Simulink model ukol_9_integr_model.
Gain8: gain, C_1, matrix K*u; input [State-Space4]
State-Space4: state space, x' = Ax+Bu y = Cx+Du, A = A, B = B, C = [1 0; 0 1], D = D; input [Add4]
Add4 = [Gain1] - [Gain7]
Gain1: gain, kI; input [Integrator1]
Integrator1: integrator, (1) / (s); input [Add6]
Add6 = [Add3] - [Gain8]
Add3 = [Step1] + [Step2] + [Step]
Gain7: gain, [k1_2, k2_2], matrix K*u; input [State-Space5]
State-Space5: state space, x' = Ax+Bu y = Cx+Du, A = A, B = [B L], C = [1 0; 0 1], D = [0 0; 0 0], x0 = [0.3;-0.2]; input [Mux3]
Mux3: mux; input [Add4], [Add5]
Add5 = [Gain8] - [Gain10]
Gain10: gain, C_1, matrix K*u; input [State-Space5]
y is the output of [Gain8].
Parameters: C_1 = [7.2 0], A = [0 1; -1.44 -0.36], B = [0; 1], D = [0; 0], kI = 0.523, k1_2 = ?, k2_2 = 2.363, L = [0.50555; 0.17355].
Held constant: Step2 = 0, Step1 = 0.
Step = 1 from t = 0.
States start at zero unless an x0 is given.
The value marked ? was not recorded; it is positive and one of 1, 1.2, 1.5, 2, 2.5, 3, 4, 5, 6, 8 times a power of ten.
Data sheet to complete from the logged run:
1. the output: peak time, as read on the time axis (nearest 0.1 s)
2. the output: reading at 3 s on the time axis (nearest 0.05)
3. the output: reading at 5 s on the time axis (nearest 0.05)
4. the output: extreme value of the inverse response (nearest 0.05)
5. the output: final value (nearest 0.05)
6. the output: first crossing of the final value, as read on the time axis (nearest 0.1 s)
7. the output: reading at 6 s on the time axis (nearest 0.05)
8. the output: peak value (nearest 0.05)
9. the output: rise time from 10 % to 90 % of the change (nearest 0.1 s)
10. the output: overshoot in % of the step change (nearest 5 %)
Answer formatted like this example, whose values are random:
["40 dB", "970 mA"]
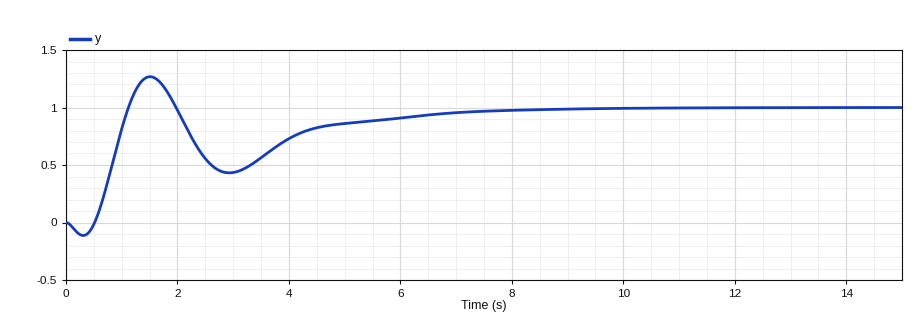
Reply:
["1.5 s", "0.45", "0.85", "-0.10", "1.00", "1.1 s", "0.90", "1.25", "0.5 s", "25 %"]
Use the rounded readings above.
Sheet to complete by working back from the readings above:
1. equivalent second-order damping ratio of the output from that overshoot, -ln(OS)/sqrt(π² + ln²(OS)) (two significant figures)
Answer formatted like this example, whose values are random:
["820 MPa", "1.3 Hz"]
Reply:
["0.40"]
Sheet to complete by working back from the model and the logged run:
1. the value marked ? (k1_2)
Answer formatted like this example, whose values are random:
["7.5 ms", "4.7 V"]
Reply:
["6"]
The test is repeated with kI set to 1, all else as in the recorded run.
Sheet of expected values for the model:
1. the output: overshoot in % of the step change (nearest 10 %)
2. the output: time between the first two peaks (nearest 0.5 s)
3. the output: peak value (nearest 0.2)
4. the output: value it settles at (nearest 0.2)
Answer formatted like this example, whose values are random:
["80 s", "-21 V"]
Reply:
["60 %", "3.0 s", "1.6", "1.0"]
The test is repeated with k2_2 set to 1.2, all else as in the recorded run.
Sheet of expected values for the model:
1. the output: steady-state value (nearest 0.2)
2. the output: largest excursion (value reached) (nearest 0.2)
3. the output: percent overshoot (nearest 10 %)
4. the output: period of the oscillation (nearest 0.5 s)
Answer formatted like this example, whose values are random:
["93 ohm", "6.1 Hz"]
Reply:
["1.0", "1.4", "40 %", "2.5 s"]
